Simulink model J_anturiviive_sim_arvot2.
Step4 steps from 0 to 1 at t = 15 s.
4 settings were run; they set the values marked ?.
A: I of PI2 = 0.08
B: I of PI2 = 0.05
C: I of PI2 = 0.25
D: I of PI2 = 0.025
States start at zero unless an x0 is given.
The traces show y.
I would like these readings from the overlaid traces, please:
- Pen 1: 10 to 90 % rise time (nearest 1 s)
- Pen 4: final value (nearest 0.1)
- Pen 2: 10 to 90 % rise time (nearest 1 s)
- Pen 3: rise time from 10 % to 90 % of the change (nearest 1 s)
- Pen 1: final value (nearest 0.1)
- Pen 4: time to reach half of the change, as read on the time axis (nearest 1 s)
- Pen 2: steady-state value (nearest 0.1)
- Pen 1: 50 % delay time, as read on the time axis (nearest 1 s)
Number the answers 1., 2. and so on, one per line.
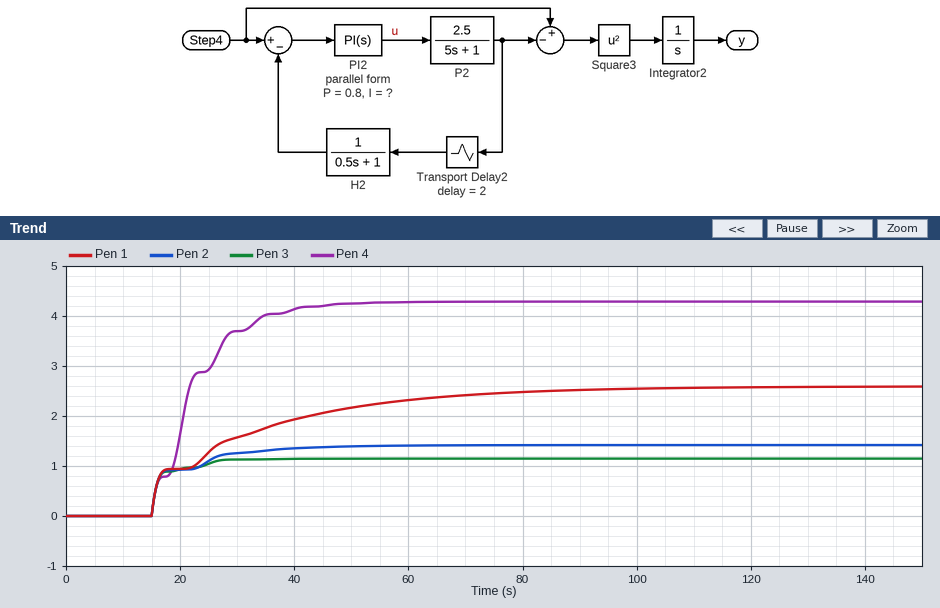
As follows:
1. 46 s
2. 4.3
3. 17 s
4. 10 s
5. 2.6
6. 21 s
7. 1.4
8. 25 s
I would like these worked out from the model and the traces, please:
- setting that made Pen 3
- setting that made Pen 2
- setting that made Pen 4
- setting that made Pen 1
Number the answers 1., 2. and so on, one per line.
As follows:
1. A
2. B
3. C
4. D
